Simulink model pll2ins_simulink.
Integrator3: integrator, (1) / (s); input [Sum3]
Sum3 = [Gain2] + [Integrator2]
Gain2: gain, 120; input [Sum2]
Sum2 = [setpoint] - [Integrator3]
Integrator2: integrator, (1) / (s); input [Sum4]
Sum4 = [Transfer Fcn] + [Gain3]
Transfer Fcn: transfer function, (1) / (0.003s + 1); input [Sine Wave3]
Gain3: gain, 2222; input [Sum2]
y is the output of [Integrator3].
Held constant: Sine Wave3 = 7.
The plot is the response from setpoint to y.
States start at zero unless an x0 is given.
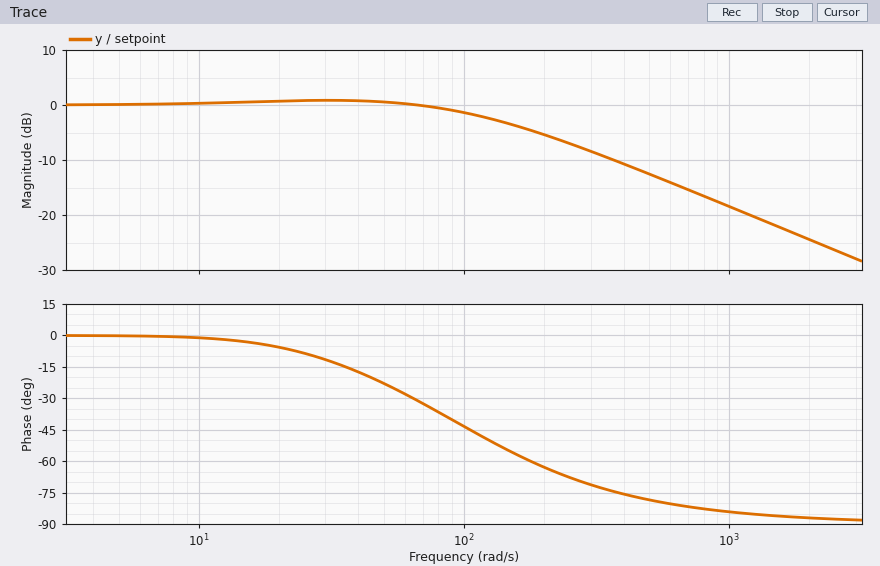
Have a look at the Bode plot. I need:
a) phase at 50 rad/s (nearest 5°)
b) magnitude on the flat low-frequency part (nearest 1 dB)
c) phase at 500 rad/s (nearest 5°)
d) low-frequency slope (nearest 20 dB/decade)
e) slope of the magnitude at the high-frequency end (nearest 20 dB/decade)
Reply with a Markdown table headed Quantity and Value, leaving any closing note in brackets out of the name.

| Quantity | Value |
|---|---|
| phase at 50 rad/s | -25° |
| magnitude on the flat low-frequency part | 0 dB |
| phase at 500 rad/s | -80° |
| low-frequency slope | 0 dB/decade |
| slope of the magnitude at the high-frequency end | -20 dB/decade |
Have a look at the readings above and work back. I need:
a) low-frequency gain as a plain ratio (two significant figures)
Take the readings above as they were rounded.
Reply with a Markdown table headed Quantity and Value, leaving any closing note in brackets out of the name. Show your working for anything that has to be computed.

| Quantity | Value |
|---|---|
| low-frequency gain as a plain ratio | 10^(0 / 20) = 1.0 |
